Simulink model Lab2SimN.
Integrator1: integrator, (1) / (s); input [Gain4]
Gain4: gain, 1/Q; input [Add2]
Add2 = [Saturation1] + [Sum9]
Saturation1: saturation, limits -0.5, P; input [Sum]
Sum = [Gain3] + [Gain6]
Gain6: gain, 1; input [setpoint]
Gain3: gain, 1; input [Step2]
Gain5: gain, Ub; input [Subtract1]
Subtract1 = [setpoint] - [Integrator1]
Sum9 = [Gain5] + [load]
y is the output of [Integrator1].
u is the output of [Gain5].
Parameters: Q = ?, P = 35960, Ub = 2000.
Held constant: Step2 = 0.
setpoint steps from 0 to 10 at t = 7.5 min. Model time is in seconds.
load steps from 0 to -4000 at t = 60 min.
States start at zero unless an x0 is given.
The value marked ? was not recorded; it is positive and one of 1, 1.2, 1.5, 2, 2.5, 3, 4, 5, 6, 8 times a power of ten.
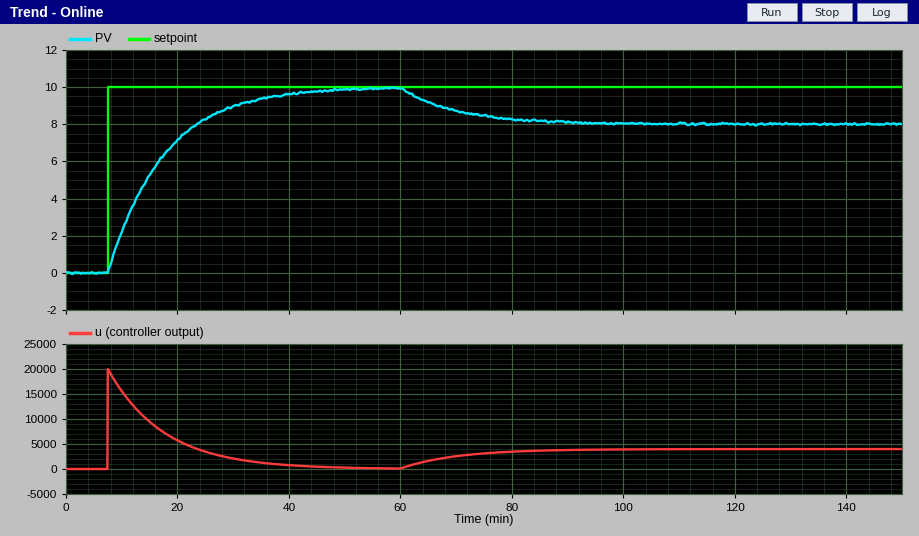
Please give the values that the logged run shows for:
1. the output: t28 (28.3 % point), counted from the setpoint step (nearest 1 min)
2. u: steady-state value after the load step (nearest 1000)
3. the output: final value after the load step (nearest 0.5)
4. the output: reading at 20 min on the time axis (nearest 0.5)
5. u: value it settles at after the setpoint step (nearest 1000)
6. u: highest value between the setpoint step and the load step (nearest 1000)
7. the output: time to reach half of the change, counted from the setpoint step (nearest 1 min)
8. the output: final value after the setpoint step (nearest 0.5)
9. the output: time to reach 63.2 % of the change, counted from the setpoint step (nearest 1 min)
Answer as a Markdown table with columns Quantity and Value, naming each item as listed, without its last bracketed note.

| Quantity | Value |
|---|---|
| the output: t28 (28.3 % point), counted from the setpoint step | 3 min |
| u: steady-state value after the load step | 4000 |
| the output: final value after the load step | 8.0 |
| the output: reading at 20 min on the time axis | 7.0 |
| u: value it settles at after the setpoint step | 0 |
| u: highest value between the setpoint step and the load step | 20000 |
| the output: time to reach half of the change, counted from the setpoint step | 7 min |
| the output: final value after the setpoint step | 10.0 |
| the output: time to reach 63.2 % of the change, counted from the setpoint step | 10 min |
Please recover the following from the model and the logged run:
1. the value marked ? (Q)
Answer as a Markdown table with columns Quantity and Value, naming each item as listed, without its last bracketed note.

| Quantity | Value |
|---|---|
| the value marked ? | 1.2e+06 |
